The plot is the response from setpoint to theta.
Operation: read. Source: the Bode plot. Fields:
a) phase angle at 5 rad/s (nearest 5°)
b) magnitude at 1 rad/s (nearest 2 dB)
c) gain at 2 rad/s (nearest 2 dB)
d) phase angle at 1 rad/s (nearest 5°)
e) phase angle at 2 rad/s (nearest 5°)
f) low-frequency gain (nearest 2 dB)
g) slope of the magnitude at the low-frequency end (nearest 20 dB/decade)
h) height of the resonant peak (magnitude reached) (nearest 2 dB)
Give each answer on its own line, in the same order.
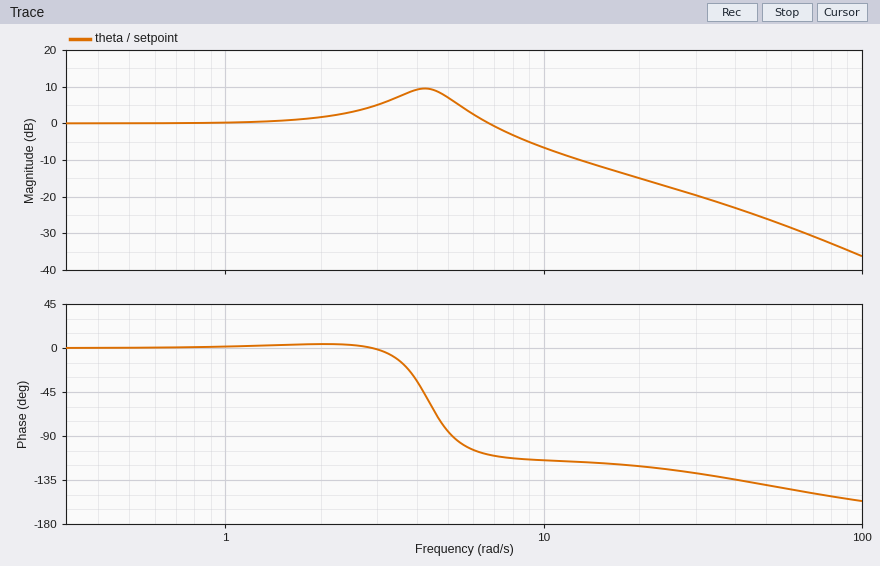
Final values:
-85°
0 dB
2 dB
0°
5°
0 dB
0 dB/decade
10 dB
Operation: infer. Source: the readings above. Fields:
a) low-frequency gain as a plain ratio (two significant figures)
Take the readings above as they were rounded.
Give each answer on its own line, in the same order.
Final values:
1.0
